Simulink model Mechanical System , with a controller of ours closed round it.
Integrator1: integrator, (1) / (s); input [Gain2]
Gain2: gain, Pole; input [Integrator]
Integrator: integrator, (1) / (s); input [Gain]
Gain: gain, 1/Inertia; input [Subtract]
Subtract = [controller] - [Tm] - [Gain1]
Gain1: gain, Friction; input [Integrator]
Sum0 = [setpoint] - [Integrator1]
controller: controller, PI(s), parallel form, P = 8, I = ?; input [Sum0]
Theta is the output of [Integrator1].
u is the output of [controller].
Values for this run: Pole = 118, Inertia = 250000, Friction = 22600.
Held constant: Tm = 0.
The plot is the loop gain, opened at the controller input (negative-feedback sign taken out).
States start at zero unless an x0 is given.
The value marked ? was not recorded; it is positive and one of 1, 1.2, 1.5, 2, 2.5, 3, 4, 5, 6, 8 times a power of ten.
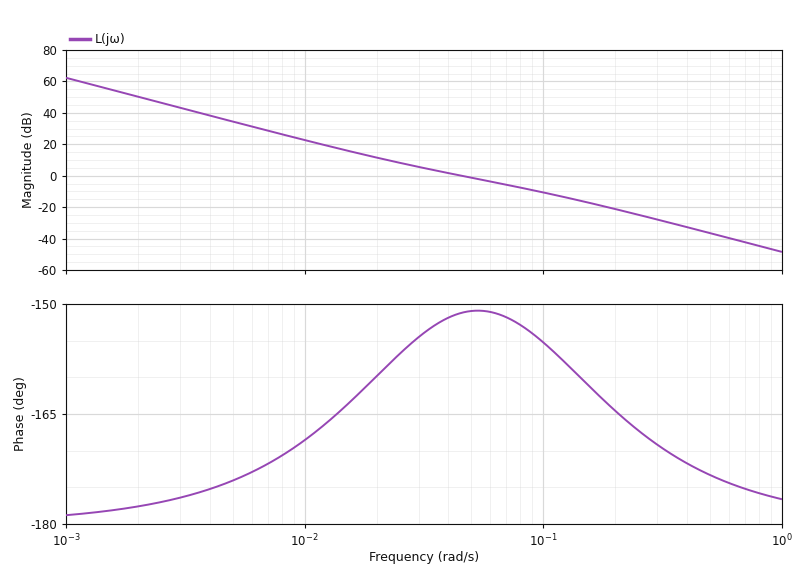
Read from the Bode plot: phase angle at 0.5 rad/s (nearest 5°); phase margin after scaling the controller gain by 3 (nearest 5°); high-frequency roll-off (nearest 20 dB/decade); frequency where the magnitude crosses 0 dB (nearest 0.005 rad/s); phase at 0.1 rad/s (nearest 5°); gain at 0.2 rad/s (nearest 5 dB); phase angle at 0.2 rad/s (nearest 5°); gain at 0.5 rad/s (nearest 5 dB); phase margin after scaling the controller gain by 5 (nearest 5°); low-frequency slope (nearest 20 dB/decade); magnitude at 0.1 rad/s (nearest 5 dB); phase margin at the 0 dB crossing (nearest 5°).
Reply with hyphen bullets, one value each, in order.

- -175°
- 25°
- -40 dB/decade
- 0.045 rad/s
- -155°
- -20 dB
- -165°
- -35 dB
- 20°
- -40 dB/decade
- -10 dB
- 30°
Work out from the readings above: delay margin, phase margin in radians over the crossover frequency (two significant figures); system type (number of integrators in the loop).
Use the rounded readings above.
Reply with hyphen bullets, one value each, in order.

- 12 s
- 2
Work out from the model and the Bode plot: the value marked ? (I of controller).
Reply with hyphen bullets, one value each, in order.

- 0.25
